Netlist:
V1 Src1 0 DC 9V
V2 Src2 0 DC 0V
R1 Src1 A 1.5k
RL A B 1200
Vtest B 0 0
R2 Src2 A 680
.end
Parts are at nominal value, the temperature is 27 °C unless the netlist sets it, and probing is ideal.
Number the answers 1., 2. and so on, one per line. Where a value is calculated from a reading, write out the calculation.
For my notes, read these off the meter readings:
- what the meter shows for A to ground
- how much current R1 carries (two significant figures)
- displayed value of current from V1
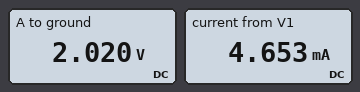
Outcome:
1. 2.020 V
2. (9 V - 2.02 V) / 1.5 kΩ = 4.7 mA
3. 4.653 mA
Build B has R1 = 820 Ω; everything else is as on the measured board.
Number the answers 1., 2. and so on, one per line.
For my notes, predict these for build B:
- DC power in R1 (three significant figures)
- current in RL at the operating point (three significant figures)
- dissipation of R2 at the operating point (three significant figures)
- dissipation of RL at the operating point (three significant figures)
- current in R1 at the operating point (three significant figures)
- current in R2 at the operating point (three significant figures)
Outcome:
1. 42.2 mW
2. 2.60 mA
3. 14.3 mW
4. 8.09 mW
5. 7.18 mA
6. 4.58 mA
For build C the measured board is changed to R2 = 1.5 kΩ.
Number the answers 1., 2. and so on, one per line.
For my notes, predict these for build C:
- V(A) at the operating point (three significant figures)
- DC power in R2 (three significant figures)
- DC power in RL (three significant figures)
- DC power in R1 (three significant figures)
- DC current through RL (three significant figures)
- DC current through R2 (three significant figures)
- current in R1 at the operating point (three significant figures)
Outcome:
1. 2.77 V
2. 5.11 mW
3. 6.39 mW
4. 25.9 mW
5. 2.31 mA
6. 1.85 mA
7. 4.15 mA
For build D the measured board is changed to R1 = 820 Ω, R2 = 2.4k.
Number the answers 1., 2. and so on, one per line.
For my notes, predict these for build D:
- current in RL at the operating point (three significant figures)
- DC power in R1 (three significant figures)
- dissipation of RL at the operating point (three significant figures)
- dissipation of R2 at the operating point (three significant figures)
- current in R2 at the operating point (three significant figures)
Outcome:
1. 3.70 mA
2. 25.3 mW
3. 16.5 mW
4. 8.23 mW
5. 1.85 mA
